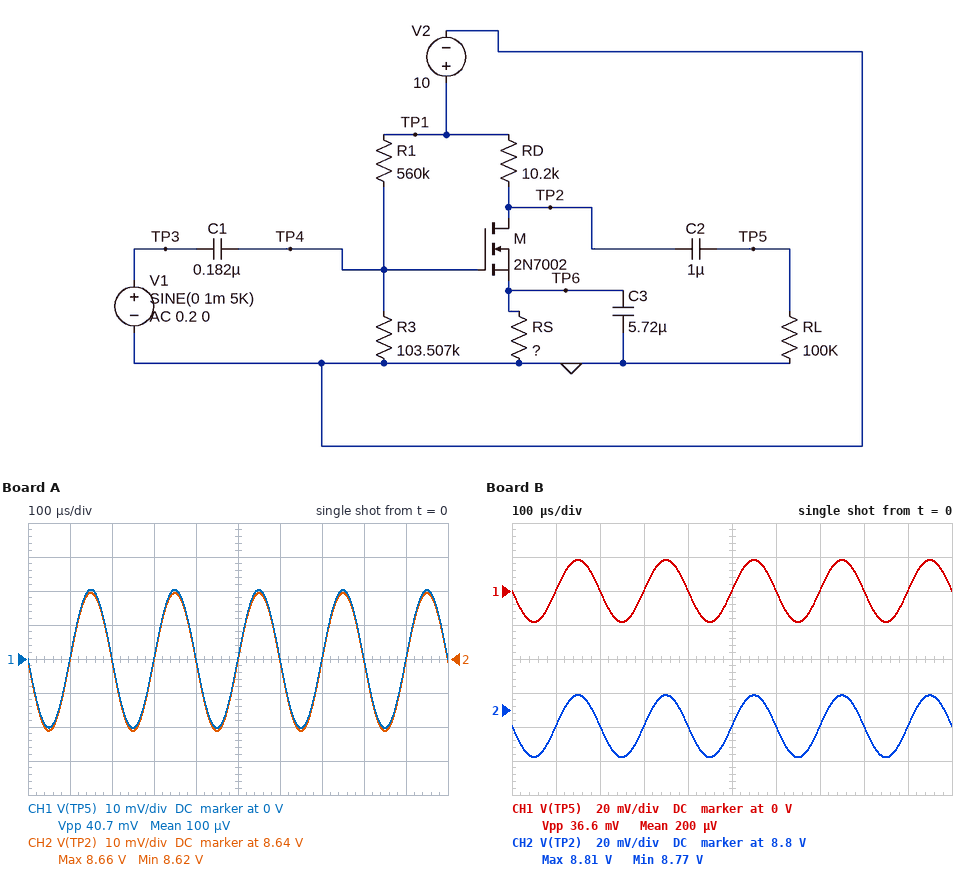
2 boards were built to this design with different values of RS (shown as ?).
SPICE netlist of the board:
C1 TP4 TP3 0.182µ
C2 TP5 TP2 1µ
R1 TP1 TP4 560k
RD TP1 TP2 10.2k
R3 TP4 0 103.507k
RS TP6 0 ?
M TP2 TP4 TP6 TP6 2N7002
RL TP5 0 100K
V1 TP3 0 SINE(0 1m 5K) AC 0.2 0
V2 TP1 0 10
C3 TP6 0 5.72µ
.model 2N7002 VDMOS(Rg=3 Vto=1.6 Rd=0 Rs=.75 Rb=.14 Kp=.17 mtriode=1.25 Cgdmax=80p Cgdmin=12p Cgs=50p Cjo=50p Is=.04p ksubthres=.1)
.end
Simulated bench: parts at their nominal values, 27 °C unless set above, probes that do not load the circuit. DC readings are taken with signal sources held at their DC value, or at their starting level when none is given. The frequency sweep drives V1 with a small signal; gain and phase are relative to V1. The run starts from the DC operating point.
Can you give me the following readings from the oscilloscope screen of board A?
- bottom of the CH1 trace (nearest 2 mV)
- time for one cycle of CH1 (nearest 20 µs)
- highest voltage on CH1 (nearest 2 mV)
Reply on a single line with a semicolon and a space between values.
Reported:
-20 mV; 200 µs; 20 mV
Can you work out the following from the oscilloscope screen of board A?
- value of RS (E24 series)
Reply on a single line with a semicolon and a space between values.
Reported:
240 Ω
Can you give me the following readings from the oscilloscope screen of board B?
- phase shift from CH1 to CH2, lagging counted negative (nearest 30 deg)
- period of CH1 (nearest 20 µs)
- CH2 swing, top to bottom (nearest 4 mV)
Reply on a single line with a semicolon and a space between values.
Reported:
0 deg; 200 µs; 36 mV
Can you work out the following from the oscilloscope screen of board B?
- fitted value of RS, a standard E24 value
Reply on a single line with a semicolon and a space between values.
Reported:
330 Ω
